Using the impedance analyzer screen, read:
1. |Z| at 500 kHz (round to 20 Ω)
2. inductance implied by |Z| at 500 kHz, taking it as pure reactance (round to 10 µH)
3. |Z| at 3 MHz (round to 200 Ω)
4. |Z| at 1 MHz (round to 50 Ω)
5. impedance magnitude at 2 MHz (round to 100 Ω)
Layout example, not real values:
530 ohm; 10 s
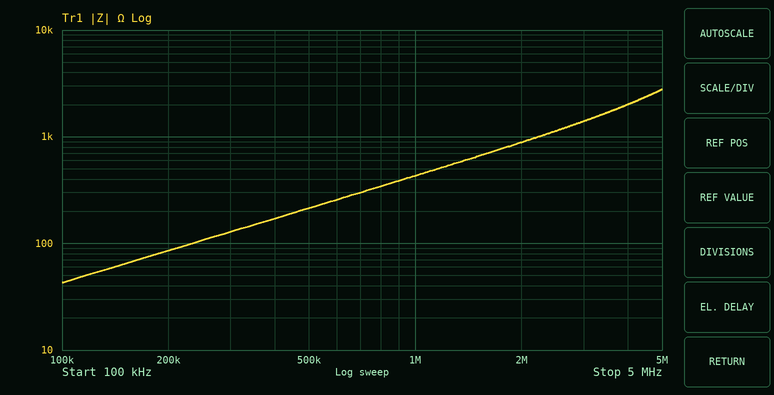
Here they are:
220 Ω; 70 µH; 1.4 kΩ; 450 Ω; 900 Ω
